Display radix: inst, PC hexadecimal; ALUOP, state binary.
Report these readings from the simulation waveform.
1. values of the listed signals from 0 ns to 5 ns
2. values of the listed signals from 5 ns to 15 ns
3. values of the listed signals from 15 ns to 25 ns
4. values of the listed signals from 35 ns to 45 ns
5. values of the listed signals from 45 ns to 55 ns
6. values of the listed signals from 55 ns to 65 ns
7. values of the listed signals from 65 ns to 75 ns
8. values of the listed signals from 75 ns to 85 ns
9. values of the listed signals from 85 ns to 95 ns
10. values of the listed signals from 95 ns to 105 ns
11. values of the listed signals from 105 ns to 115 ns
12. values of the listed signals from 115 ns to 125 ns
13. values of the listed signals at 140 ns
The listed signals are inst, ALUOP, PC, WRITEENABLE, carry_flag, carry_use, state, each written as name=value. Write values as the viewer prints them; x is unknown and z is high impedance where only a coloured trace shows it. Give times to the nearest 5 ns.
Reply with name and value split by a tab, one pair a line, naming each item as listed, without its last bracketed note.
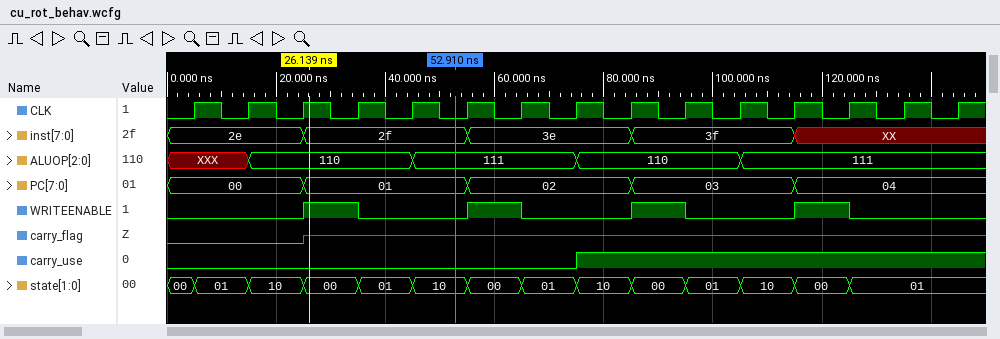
values of the listed signals from 0 ns to 5 ns	inst=2e, ALUOP=XXX, PC=00, WRITEENABLE=0, carry_flag=0, carry_use=0, state=00
values of the listed signals from 5 ns to 15 ns	inst=2e, ALUOP=XXX, PC=00, WRITEENABLE=0, carry_flag=0, carry_use=0, state=01
values of the listed signals from 15 ns to 25 ns	inst=2e, ALUOP=110, PC=00, WRITEENABLE=0, carry_flag=0, carry_use=0, state=10
values of the listed signals from 35 ns to 45 ns	inst=2f, ALUOP=110, PC=01, WRITEENABLE=0, carry_flag=z, carry_use=0, state=01
values of the listed signals from 45 ns to 55 ns	inst=2f, ALUOP=111, PC=01, WRITEENABLE=0, carry_flag=z, carry_use=0, state=10
values of the listed signals from 55 ns to 65 ns	inst=3e, ALUOP=111, PC=02, WRITEENABLE=1, carry_flag=z, carry_use=0, state=00
values of the listed signals from 65 ns to 75 ns	inst=3e, ALUOP=111, PC=02, WRITEENABLE=0, carry_flag=z, carry_use=0, state=01
values of the listed signals from 75 ns to 85 ns	inst=3e, ALUOP=110, PC=02, WRITEENABLE=0, carry_flag=z, carry_use=1, state=10
values of the listed signals from 85 ns to 95 ns	inst=3f, ALUOP=110, PC=03, WRITEENABLE=1, carry_flag=z, carry_use=1, state=00
values of the listed signals from 95 ns to 105 ns	inst=3f, ALUOP=110, PC=03, WRITEENABLE=0, carry_flag=z, carry_use=1, state=01
values of the listed signals from 105 ns to 115 ns	inst=3f, ALUOP=111, PC=03, WRITEENABLE=0, carry_flag=z, carry_use=1, state=10
values of the listed signals from 115 ns to 125 ns	inst=XX, ALUOP=111, PC=04, WRITEENABLE=1, carry_flag=z, carry_use=1, state=00
values of the listed signals at 140 ns	inst=XX, ALUOP=111, PC=04, WRITEENABLE=0, carry_flag=z, carry_use=1, state=01
